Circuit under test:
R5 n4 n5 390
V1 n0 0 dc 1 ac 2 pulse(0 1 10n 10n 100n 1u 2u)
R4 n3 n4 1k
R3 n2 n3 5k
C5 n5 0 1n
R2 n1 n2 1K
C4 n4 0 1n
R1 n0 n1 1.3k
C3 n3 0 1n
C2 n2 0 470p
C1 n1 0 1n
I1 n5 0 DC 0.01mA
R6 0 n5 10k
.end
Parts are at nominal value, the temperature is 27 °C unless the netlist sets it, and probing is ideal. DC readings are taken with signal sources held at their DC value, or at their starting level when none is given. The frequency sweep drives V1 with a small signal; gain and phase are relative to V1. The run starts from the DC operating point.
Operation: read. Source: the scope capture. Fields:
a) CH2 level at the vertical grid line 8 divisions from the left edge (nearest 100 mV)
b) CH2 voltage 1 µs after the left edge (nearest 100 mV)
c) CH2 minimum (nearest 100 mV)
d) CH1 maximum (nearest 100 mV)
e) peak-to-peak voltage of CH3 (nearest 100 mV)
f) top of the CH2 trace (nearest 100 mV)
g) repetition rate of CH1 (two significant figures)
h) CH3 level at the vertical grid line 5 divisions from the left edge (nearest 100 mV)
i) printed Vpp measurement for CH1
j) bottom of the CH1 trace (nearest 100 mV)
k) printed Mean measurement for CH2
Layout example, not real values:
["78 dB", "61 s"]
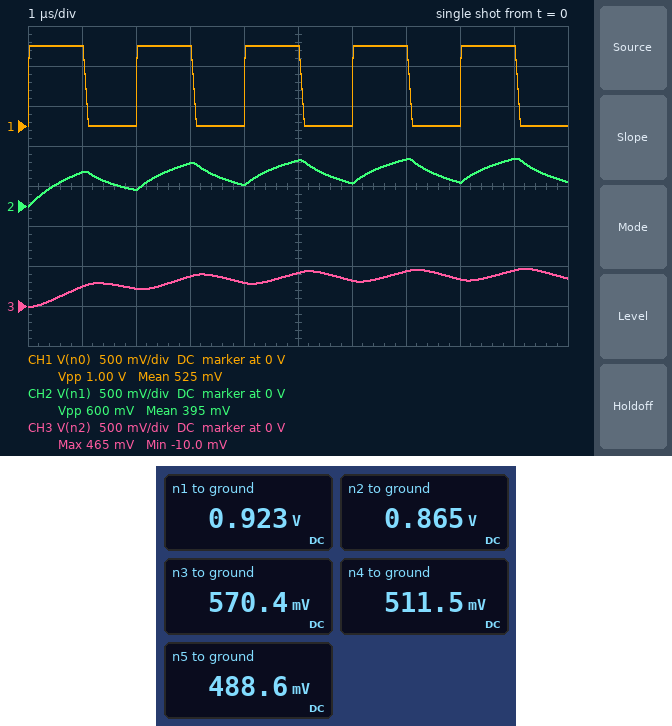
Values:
["300 mV", "400 mV", "0 V", "1.0 V", "500 mV", "600 mV", "500 kHz", "400 mV", "1.00 V", "0 V", "395 mV"]
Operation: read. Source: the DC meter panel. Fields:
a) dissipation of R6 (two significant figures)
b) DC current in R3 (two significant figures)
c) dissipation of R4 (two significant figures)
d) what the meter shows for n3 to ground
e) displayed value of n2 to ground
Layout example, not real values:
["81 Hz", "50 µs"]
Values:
["24 µW", "59 µA", "3.5 µW", "570.4 mV", "0.865 V"]
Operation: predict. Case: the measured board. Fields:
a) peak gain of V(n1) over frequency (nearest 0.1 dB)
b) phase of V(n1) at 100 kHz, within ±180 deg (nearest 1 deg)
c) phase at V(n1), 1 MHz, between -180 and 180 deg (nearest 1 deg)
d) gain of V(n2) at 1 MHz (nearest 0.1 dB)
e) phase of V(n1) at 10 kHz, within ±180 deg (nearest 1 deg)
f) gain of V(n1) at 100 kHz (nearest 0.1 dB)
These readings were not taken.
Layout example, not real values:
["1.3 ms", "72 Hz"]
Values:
["-0.6 dB", "-41 deg", "-76 deg", "-29.0 dB", "-9 deg", "-4.5 dB"]
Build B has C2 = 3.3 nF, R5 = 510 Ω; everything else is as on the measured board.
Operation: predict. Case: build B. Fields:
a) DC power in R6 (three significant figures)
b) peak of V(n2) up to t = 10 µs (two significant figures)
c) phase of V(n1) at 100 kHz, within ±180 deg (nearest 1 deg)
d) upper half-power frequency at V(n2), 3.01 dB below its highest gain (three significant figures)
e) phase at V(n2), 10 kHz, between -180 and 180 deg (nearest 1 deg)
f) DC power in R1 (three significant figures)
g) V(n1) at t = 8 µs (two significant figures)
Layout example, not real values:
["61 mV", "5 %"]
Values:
["23.5 µW", "310 mV", "-32 deg", "15.8 kHz", "-30 deg", "4.45 µW", "220 mV"]
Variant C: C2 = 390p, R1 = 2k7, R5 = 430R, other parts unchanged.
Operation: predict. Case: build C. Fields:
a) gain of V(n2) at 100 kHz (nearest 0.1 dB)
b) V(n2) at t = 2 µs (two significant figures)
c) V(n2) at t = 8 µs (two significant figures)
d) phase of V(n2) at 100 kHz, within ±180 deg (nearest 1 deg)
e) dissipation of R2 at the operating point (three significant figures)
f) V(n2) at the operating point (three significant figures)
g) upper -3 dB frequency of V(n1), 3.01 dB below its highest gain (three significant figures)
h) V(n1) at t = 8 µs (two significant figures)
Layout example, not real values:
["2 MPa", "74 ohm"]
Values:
["-10.2 dB", "140 mV", "280 mV", "-68 deg", "2.99 µW", "798 mV", "33.9 kHz", "290 mV"]
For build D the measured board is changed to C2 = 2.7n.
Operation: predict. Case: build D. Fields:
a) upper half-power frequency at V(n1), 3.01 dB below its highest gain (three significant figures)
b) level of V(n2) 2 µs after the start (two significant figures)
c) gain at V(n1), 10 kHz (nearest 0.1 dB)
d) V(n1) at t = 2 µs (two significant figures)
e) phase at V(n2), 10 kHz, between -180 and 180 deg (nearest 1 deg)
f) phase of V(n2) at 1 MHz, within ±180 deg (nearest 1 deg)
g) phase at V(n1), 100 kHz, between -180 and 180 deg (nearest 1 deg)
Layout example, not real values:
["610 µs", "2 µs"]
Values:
["28.2 kHz", "100 mV", "-1.6 dB", "120 mV", "-27 deg", "-160 deg", "-34 deg"]
